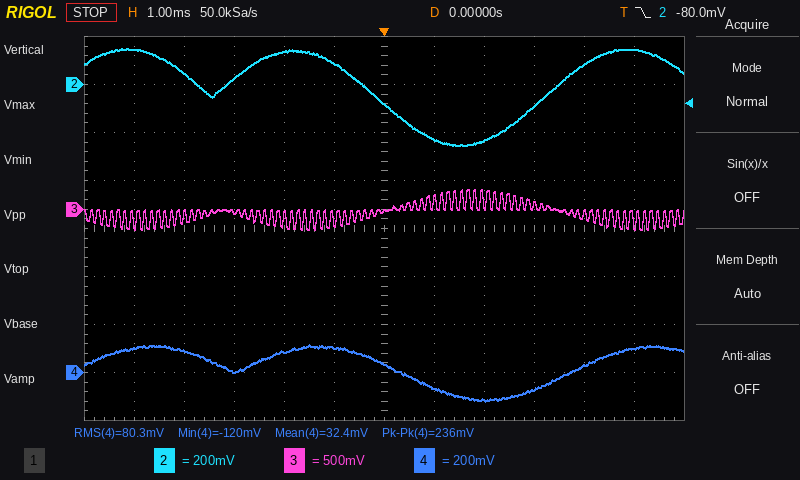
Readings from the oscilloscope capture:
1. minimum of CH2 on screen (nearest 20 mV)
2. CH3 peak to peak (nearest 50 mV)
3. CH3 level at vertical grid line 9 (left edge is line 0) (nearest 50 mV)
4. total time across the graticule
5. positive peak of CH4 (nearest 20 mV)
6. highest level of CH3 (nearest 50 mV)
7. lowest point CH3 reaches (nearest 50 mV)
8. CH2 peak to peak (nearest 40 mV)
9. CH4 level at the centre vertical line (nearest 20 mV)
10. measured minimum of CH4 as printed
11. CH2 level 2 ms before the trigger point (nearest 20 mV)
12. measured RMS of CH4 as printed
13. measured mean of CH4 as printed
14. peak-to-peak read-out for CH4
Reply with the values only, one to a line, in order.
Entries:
-260 mV
400 mV
50 mV
12 ms
120 mV
200 mV
-200 mV
400 mV
40 mV
-120 mV
140 mV
80.3 mV
32.4 mV
236 mV
